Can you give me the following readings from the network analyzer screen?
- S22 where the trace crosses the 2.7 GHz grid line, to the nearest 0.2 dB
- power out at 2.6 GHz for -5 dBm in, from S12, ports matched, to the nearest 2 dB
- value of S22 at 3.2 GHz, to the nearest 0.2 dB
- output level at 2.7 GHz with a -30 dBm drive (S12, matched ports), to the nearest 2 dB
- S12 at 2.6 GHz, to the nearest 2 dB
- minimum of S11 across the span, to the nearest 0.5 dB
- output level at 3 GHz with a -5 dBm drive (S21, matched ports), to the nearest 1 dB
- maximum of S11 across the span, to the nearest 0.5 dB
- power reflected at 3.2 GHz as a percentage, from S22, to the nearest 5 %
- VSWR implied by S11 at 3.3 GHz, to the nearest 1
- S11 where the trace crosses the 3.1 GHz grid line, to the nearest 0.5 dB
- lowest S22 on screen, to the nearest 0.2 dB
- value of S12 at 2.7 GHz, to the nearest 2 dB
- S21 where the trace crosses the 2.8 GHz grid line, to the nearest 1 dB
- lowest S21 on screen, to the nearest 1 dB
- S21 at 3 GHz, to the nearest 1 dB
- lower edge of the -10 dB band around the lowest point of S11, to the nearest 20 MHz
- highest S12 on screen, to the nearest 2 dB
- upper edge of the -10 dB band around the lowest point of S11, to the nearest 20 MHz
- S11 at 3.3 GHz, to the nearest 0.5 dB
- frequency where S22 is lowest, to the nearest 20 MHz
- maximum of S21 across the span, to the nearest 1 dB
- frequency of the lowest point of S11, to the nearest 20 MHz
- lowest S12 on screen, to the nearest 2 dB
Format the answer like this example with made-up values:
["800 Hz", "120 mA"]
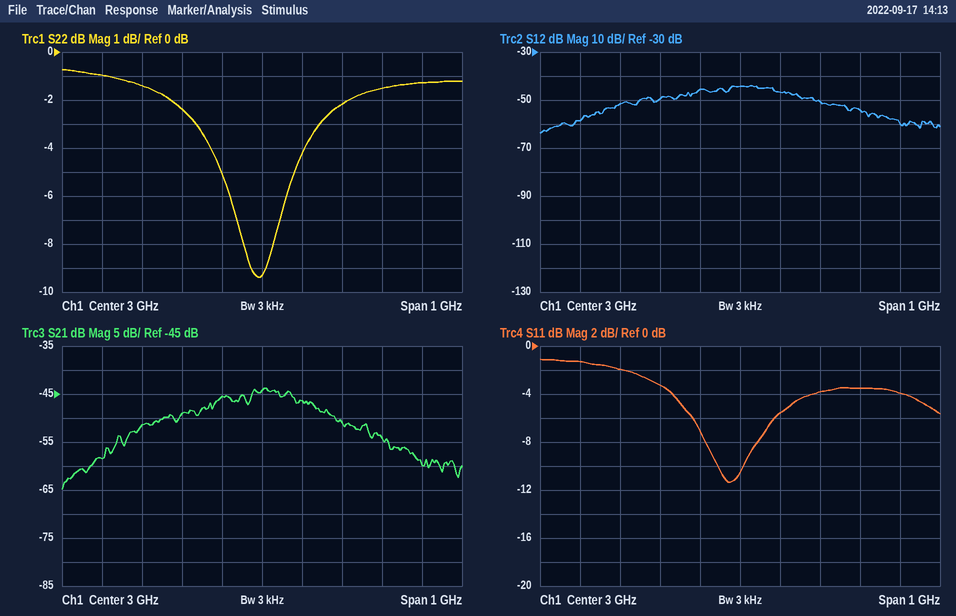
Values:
["-1.4 dB", "-64 dBm", "-2.2 dB", "-82 dBm", "-58 dB", "-11.5 dB", "-49 dBm", "-1.0 dB", "60 %", "5", "-5.5 dB", "-9.4 dB", "-52 dB", "-49 dB", "-65 dB", "-44 dB", "2.94 GHz", "-44 dB", "3.00 GHz", "-3.5 dB", "3.00 GHz", "-44 dB", "2.98 GHz", "-64 dB"]
